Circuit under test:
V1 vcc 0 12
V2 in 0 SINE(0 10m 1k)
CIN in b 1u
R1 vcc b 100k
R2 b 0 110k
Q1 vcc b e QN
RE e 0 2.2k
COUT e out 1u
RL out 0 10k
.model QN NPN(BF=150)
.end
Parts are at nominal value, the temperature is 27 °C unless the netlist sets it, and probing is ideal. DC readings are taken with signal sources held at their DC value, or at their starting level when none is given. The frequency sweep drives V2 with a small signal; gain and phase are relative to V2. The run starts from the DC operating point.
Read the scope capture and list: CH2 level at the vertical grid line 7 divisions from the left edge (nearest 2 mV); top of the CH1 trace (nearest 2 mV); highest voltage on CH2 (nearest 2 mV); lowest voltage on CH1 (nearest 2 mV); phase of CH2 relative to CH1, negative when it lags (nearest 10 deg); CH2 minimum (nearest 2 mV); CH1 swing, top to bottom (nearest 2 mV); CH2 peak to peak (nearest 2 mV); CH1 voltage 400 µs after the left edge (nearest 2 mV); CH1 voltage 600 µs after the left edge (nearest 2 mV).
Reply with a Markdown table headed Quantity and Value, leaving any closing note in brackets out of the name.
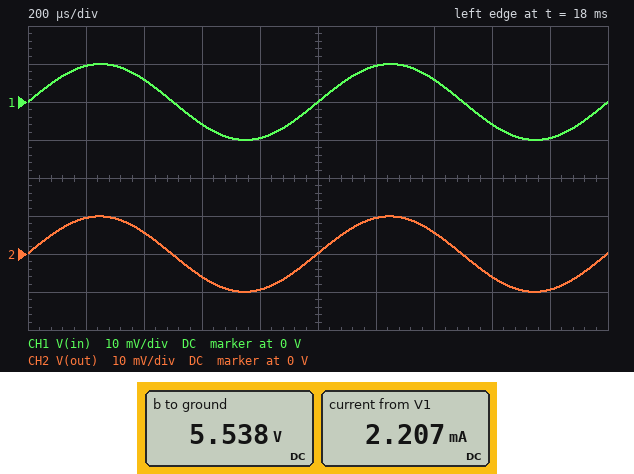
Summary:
| Quantity | Value |
|---|---|
| CH2 level at the vertical grid line 7 divisions from the left edge | 6 mV |
| top of the CH1 trace | 10 mV |
| highest voltage on CH2 | 10 mV |
| lowest voltage on CH1 | -10 mV |
| phase of CH2 relative to CH1, negative when it lags | 0 deg |
| CH2 minimum | -10 mV |
| CH1 swing, top to bottom | 20 mV |
| CH2 peak to peak | 20 mV |
| CH1 voltage 400 µs after the left edge | 6 mV |
| CH1 voltage 600 µs after the left edge | -6 mV |
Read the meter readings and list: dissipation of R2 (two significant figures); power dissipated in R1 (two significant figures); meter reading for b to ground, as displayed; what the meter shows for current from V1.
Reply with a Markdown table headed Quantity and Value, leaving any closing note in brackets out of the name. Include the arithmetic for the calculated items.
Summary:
| Quantity | Value |
|---|---|
| dissipation of R2 | (5.538 V)^2 / 110 kΩ = 280 µW |
| power dissipated in R1 | (12 V - 5.538 V)^2 / 100 kΩ = 420 µW |
| meter reading for b to ground, as displayed | 5.538 V |
| what the meter shows for current from V1 | 2.207 mA |
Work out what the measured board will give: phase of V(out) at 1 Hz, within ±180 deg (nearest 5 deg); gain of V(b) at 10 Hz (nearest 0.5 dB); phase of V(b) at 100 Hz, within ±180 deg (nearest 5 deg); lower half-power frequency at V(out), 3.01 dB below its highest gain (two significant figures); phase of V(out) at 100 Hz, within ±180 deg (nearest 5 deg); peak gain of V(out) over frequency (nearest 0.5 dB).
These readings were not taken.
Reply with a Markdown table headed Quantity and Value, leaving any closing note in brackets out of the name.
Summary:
| Quantity | Value |
|---|---|
| phase of V(out) at 1 Hz, within ±180 deg | 160 deg |
| gain of V(b) at 10 Hz | -0.5 dB |
| phase of V(b) at 100 Hz, within ±180 deg | 0 deg |
| lower half-power frequency at V(out), 3.01 dB below its highest gain | 17 Hz |
| phase of V(out) at 100 Hz, within ±180 deg | 10 deg |
| peak gain of V(out) over frequency | 0 dB |
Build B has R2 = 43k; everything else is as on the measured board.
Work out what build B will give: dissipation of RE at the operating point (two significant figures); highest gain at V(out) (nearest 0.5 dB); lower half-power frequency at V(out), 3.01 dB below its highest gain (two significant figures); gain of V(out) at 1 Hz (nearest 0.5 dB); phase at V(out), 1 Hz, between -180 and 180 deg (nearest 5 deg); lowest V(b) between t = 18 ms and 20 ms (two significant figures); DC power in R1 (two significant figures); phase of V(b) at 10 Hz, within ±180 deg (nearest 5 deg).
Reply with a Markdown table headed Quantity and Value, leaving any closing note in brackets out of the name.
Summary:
| Quantity | Value |
|---|---|
| dissipation of RE at the operating point | 3.1 mW |
| highest gain at V(out) | 0 dB |
| lower half-power frequency at V(out), 3.01 dB below its highest gain | 18 Hz |
| gain of V(out) at 1 Hz | -39.5 dB |
| phase at V(out), 1 Hz, between -180 and 180 deg | 165 deg |
| lowest V(b) between t = 18 ms and 20 ms | 3.4 V |
| DC power in R1 | 740 µW |
| phase of V(b) at 10 Hz, within ±180 deg | 30 deg |
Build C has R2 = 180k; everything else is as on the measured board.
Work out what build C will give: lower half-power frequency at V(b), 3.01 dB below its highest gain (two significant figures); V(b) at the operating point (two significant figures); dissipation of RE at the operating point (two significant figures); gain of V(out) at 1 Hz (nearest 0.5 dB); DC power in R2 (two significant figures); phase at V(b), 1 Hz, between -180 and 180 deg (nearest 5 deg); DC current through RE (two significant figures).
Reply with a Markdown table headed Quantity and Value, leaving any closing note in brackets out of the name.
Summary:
| Quantity | Value |
|---|---|
| lower half-power frequency at V(b), 3.01 dB below its highest gain | 3.0 Hz |
| V(b) at the operating point | 6.6 V |
| dissipation of RE at the operating point | 15 mW |
| gain of V(out) at 1 Hz | -34.0 dB |
| DC power in R2 | 240 µW |
| phase at V(b), 1 Hz, between -180 and 180 deg | 70 deg |
| DC current through RE | 2.6 mA |
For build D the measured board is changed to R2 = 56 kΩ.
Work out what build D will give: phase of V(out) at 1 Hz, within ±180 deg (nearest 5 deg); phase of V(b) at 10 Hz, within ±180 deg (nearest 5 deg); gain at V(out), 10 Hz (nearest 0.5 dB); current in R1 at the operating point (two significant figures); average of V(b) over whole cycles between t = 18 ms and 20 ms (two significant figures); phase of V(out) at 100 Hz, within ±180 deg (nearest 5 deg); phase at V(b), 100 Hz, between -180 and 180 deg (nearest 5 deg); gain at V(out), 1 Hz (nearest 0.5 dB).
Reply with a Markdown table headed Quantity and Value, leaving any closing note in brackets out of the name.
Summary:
| Quantity | Value |
|---|---|
| phase of V(out) at 1 Hz, within ±180 deg | 165 deg |
| phase of V(b) at 10 Hz, within ±180 deg | 25 deg |
| gain at V(out), 10 Hz | -6.5 dB |
| current in R1 at the operating point | 80 µA |
| average of V(b) over whole cycles between t = 18 ms and 20 ms | 4.0 V |
| phase of V(out) at 100 Hz, within ±180 deg | 10 deg |
| phase at V(b), 100 Hz, between -180 and 180 deg | 5 deg |
| gain at V(out), 1 Hz | -38.0 dB |
